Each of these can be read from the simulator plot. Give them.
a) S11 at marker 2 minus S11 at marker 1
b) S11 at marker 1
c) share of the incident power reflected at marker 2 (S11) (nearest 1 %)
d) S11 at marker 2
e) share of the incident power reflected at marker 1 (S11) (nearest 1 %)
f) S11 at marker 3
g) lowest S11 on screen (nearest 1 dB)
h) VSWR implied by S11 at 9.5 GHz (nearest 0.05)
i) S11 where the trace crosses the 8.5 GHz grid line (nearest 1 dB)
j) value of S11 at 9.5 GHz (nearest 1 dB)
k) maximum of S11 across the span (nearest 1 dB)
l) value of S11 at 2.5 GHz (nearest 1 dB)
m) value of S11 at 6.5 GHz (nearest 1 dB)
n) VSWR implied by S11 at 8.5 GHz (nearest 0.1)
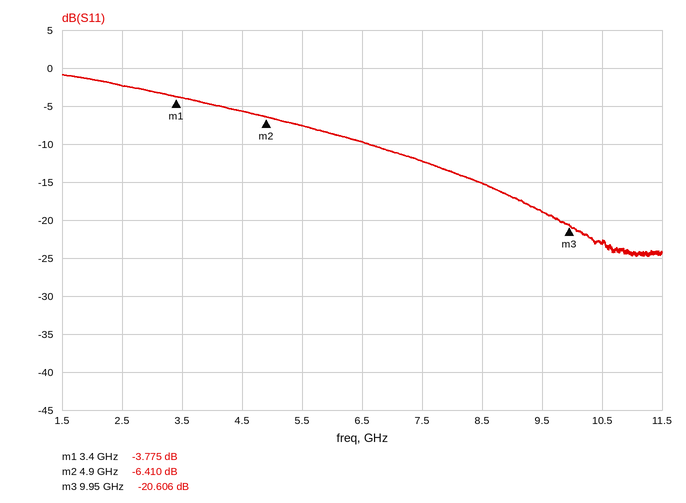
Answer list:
-2.635 dB
-3.775 dB
23 %
-6.410 dB
42 %
-20.606 dB
-25 dB
1.25
-15 dB
-19 dB
-1 dB
-2 dB
-10 dB
1.4
